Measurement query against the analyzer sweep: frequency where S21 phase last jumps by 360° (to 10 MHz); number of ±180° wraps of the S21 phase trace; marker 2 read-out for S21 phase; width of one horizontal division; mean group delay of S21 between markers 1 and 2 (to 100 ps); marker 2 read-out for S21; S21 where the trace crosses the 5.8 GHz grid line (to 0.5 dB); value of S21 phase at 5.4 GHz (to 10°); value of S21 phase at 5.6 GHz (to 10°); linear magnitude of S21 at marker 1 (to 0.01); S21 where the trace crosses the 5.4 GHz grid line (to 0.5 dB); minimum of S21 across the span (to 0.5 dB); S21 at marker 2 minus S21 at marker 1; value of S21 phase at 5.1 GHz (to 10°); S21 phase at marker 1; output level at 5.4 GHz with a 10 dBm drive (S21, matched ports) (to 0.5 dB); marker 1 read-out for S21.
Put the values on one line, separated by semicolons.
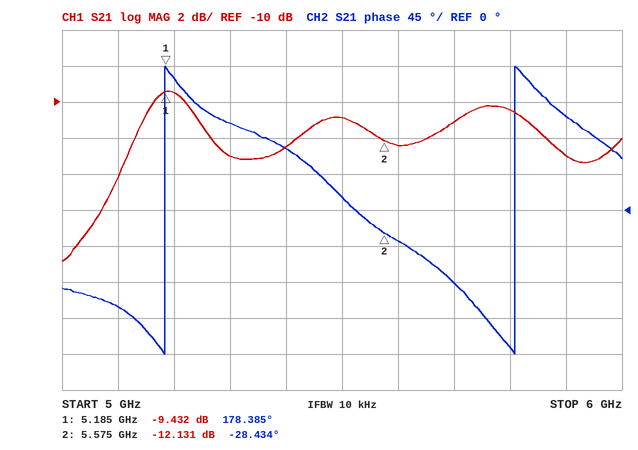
5.81 GHz; 2; -28.434°; 100 MHz; 1.5 ns; -12.131 dB; -10.5 dB; 80°; -40°; 0.34; -12.5 dB; -19.0 dB; -2.699 dB; -120°; 178.385°; -2.5 dBm; -9.432 dB
